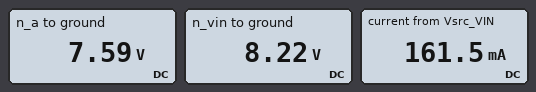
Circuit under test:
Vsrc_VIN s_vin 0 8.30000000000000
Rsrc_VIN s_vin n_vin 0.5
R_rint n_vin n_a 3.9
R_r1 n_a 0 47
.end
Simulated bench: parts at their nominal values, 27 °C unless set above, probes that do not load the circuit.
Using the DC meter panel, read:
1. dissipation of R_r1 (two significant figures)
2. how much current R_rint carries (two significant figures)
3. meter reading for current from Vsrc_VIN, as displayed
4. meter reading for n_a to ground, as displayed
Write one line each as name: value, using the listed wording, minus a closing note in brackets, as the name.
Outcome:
dissipation of R_r1: 1.2 W
how much current R_rint carries: 160 mA
meter reading for current from Vsrc_VIN, as displayed: 161.5 mA
meter reading for n_a to ground, as displayed: 7.59 V
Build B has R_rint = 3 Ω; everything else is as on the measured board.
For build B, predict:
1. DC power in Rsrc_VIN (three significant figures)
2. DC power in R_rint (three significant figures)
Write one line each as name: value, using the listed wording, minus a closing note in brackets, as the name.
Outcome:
DC power in Rsrc_VIN: 13.5 mW
DC power in R_rint: 81.0 mW
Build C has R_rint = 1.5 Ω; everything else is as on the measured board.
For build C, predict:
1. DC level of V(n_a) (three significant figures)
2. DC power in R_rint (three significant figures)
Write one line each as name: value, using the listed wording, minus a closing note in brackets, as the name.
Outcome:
DC level of V(n_a): 7.96 V
DC power in R_rint: 43.0 mW
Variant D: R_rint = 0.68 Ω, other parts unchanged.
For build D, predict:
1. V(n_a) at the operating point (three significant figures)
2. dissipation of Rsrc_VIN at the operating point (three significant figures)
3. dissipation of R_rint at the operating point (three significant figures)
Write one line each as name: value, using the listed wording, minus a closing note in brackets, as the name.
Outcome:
V(n_a) at the operating point: 8.10 V
dissipation of Rsrc_VIN at the operating point: 14.8 mW
dissipation of R_rint at the operating point: 20.2 mW
